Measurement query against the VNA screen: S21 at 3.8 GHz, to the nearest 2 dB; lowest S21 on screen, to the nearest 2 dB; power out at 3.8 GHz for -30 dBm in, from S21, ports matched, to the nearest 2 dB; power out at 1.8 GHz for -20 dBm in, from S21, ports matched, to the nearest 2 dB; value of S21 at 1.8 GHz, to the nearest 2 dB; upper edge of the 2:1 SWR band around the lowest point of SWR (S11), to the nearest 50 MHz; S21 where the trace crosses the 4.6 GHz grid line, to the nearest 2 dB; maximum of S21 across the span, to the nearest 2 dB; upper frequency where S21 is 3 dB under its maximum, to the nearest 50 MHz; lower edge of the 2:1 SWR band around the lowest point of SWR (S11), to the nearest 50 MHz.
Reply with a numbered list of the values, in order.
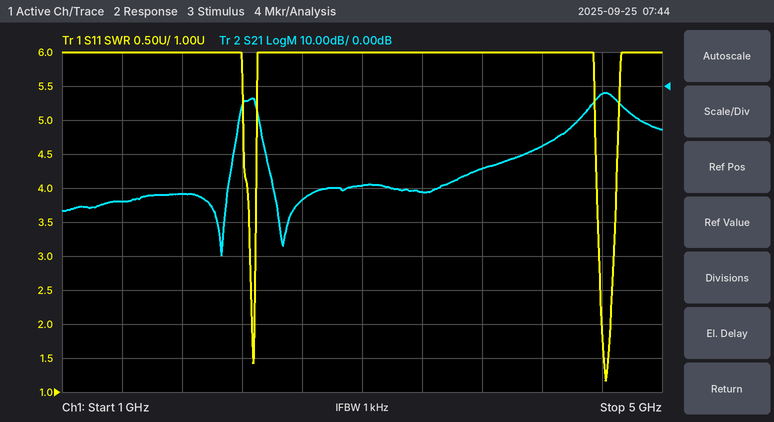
1. -24 dB
2. -50 dB
3. -54 dBm
4. -52 dBm
5. -32 dB
6. 4.65 GHz
7. -2 dB
8. -2 dB
9. 4.70 GHz
10. 4.60 GHz
